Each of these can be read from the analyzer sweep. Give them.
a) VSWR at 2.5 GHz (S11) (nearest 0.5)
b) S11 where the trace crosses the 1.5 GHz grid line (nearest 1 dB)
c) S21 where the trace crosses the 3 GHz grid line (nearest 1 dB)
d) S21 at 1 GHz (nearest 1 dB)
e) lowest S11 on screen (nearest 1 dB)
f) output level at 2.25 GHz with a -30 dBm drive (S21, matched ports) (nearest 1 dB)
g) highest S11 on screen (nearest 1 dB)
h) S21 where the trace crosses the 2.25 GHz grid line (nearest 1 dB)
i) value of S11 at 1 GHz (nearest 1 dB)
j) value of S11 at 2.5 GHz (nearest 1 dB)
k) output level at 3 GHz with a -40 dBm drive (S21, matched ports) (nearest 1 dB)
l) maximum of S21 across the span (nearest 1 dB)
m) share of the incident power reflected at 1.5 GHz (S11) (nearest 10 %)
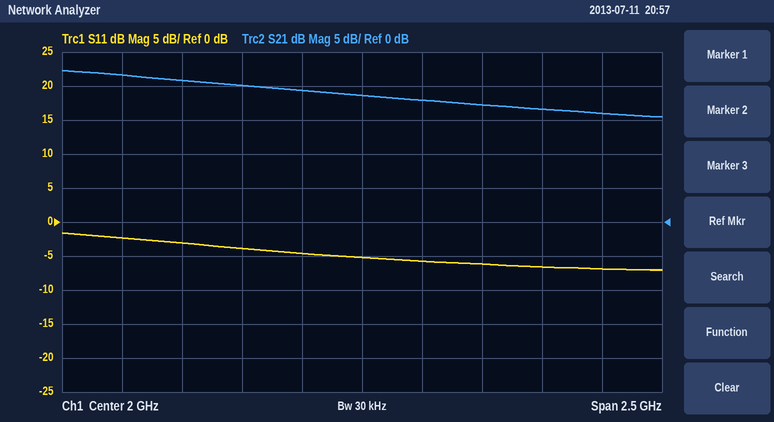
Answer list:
3.0
-4 dB
16 dB
22 dB
-7 dB
-12 dBm
-2 dB
18 dB
-2 dB
-6 dB
-24 dBm
22 dB
40 %
